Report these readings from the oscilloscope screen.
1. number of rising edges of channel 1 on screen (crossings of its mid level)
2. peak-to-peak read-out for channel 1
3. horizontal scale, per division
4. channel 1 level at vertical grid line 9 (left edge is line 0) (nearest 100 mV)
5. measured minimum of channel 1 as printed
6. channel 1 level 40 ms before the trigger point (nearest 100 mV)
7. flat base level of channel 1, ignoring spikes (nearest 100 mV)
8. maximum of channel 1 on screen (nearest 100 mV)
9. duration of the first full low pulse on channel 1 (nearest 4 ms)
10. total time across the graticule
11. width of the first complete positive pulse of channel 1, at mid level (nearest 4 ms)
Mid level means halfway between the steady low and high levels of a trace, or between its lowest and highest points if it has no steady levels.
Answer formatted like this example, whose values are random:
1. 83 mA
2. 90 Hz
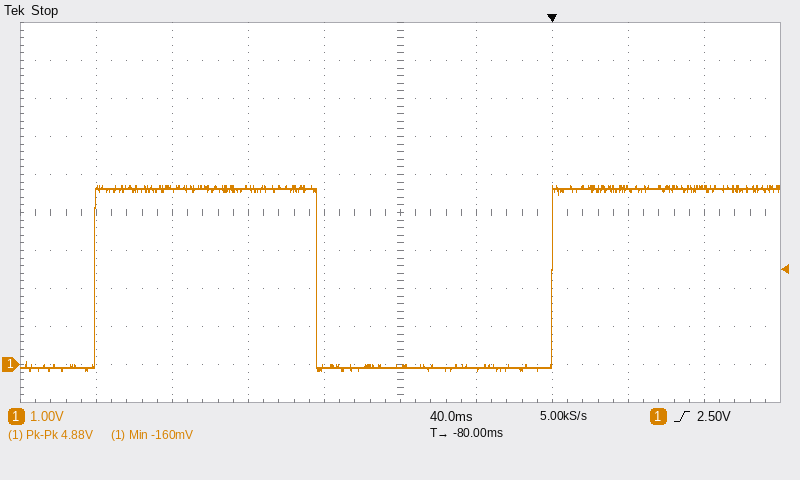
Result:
1. 2
2. 4.88 V
3. 40 ms
4. 4.6 V
5. -160 mV
6. -100 mV
7. -100 mV
8. 4.7 V
9. 124 ms
10. 400 ms
11. 116 ms
